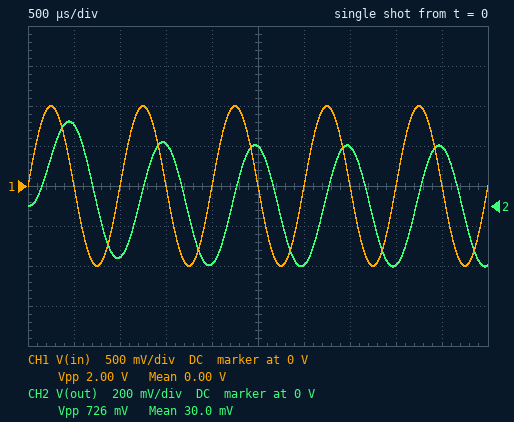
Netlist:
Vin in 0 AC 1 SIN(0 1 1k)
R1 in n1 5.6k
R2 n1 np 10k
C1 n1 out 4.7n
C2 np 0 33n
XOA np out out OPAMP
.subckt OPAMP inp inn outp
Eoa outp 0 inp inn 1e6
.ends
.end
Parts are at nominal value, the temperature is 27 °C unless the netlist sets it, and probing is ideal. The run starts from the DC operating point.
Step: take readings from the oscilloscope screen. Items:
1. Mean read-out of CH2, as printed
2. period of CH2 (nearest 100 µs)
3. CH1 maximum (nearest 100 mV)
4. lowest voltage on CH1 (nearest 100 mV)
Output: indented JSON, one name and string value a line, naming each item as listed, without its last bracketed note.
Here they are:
{
  "Mean read-out of CH2, as printed": "30.0 mV",
  "period of CH2": "1.0 ms",
  "CH1 maximum": "1.0 V",
  "lowest voltage on CH1": "-1.0 V"
}
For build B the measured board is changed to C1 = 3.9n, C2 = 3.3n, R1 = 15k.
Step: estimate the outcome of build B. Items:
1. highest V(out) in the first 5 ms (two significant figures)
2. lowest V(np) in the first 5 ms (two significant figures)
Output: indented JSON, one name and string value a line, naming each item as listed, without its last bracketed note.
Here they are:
{
  "highest V(out) in the first 5 ms": "940 mV",
  "lowest V(np) in the first 5 ms": "-940 mV"
}
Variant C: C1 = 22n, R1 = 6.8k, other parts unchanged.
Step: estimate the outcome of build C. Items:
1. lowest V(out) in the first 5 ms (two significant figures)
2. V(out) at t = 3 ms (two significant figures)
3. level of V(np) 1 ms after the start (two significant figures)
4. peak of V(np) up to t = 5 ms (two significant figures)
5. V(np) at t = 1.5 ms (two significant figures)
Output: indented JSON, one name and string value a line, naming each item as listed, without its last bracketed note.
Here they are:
{
  "lowest V(out) in the first 5 ms": "-280 mV",
  "V(out) at t = 3 ms": "-270 mV",
  "level of V(np) 1 ms after the start": "-220 mV",
  "peak of V(np) up to t = 5 ms": "400 mV",
  "V(np) at t = 1.5 ms": "280 mV"
}
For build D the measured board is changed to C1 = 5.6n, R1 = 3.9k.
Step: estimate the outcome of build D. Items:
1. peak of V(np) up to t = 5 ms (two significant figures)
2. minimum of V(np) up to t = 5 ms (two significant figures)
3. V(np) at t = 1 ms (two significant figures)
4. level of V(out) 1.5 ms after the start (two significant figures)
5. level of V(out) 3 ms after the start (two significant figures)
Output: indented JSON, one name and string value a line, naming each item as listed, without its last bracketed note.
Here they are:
{
  "peak of V(np) up to t = 5 ms": "460 mV",
  "minimum of V(np) up to t = 5 ms": "-340 mV",
  "V(np) at t = 1 ms": "-290 mV",
  "level of V(out) 1.5 ms after the start": "340 mV",
  "level of V(out) 3 ms after the start": "-330 mV"
}
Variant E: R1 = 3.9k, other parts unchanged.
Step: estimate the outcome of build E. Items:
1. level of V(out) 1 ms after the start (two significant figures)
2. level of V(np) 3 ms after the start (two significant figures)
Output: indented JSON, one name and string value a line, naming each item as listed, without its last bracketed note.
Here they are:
{
  "level of V(out) 1 ms after the start": "-290 mV",
  "level of V(np) 3 ms after the start": "-320 mV"
}
